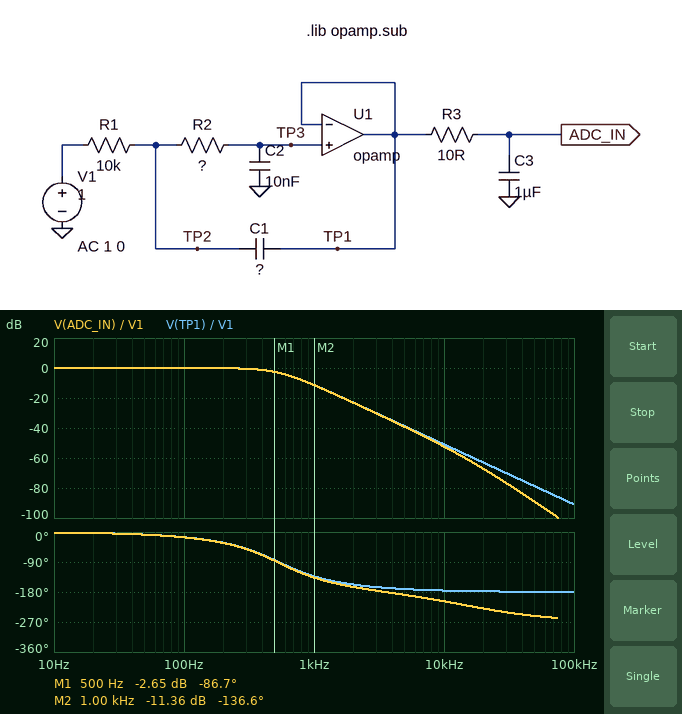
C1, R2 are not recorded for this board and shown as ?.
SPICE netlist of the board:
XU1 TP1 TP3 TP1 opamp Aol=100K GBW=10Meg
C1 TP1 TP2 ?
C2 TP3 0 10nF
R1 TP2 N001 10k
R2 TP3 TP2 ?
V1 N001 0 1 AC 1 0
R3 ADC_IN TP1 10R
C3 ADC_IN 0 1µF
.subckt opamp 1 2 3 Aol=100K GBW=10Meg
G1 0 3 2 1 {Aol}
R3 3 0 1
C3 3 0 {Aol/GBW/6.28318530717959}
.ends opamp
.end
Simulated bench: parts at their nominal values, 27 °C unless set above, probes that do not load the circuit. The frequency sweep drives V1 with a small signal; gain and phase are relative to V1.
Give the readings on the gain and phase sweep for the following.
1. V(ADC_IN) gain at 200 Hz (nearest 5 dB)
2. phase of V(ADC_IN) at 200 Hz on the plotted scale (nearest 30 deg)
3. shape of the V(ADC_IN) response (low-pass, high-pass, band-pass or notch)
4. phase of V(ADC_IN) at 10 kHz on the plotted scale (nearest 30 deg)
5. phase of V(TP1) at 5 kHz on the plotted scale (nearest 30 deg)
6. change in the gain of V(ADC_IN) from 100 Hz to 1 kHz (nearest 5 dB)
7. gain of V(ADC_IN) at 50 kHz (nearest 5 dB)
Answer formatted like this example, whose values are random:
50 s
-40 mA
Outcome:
0 dB
-30 deg
low-pass
-210 deg
-180 deg
-10 dB
-90 dB
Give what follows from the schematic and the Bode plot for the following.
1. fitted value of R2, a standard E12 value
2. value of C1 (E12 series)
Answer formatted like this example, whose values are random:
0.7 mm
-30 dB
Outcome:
33 kΩ
27 nF
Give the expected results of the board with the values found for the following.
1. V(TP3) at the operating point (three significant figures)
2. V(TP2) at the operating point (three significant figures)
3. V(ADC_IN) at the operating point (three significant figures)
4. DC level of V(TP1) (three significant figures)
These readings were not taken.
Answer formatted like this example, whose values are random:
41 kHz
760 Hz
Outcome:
1.00 V
1.00 V
1.00 V
1.00 V
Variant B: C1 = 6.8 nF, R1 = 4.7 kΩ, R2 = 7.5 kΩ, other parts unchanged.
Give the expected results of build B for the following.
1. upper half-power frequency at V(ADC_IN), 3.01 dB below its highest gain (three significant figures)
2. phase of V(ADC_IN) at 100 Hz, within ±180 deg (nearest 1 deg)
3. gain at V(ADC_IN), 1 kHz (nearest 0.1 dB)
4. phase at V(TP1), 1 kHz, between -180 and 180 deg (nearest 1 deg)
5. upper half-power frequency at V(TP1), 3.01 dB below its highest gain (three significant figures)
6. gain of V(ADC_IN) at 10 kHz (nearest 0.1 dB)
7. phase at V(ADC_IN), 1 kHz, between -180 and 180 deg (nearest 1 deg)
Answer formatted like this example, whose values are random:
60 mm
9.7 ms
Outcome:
1.53 kHz
-5 deg
-1.5 dB
-40 deg
1.54 kHz
-22.6 dB
-44 deg
